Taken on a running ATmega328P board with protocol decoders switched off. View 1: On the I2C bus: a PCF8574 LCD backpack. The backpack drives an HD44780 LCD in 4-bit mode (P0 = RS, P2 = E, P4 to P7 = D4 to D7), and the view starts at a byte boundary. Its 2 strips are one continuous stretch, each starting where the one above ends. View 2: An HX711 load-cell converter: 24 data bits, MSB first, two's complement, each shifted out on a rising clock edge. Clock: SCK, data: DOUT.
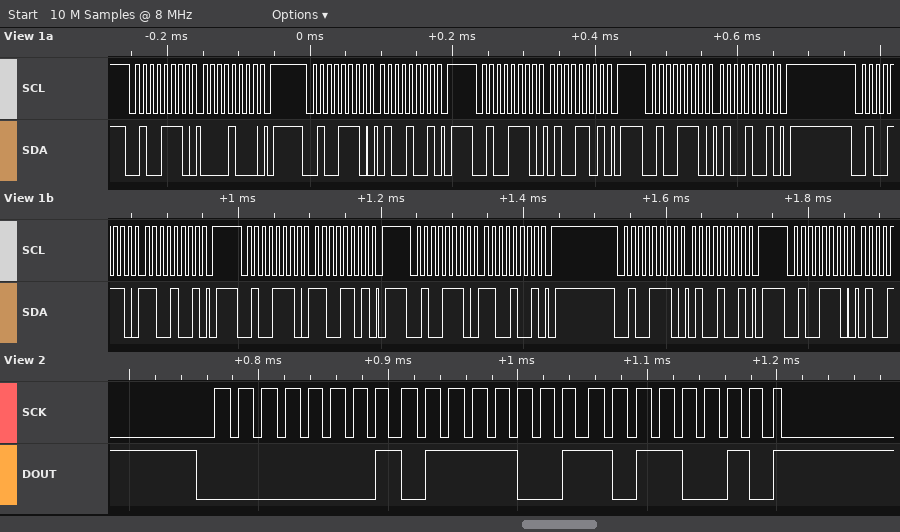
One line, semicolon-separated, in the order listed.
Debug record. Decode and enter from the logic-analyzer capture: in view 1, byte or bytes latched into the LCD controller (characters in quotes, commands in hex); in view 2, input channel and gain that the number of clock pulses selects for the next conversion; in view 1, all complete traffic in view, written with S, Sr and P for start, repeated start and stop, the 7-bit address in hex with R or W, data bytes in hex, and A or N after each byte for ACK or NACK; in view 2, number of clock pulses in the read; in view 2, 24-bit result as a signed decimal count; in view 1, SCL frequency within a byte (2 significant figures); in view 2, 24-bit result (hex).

'L'; channel A, gain 128; S 27W A 08 A P S 27W A 49 A P S 27W A 4D A P S 27W A 49 A P S 27W A C9 A P S 27W A CD A P S 27W A C9 A P S 27W A 49 A P S 27W A; 25; 96690; 100 kHz; 0x0179B2
